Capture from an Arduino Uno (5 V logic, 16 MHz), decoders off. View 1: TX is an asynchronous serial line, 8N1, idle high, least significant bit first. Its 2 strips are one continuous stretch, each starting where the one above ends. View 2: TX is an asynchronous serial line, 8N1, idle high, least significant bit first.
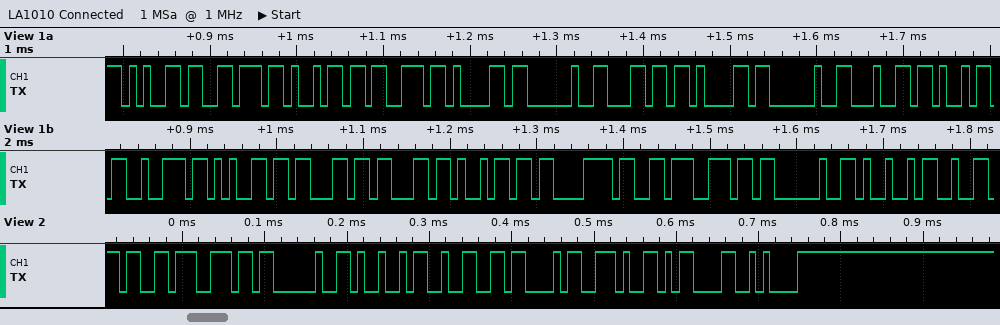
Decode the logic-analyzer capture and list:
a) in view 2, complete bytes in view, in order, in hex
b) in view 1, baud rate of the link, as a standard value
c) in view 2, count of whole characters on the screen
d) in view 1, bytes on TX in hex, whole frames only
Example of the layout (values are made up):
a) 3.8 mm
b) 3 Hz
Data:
a) B3 6E 20 49 32 43 2E 0D 0A
b) 115200 baud
c) 9
d) 65 76 69 73 61 20 6C 61 20 64 69 72 65 63 63 69 C3 B3 6E 20 49
